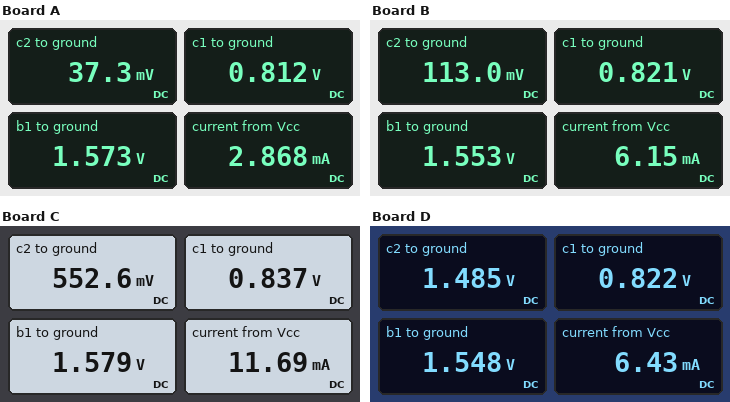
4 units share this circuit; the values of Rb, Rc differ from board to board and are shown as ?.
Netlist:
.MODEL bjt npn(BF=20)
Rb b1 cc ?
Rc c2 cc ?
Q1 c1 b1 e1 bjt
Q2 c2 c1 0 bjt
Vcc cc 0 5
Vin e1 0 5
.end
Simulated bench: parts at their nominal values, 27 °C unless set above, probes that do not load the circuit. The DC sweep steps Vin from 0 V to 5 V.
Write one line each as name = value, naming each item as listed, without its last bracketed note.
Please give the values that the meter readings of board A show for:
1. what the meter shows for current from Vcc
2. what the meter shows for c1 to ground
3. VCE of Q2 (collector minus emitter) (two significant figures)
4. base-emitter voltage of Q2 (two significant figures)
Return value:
what the meter shows for current from Vcc = 2.868 mA
what the meter shows for c1 to ground = 0.812 V
VCE of Q2 (collector minus emitter) = 37 mV
base-emitter voltage of Q2 = 810 mV
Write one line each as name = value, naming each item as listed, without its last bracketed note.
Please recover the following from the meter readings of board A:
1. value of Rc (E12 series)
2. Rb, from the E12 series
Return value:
value of Rc = 2.2 kΩ
Rb, from the E12 series = 5.6 kΩ
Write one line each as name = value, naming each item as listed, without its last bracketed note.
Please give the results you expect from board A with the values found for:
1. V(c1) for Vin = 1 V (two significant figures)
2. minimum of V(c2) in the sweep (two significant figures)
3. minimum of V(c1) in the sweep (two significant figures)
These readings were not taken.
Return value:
V(c1) for Vin = 1 V = 810 mV
minimum of V(c2) in the sweep = 37 mV
minimum of V(c1) in the sweep = 18 mV
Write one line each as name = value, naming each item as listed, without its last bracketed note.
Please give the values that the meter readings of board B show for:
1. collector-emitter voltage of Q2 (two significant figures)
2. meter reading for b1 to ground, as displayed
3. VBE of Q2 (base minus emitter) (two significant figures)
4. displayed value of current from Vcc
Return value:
collector-emitter voltage of Q2 = 110 mV
meter reading for b1 to ground, as displayed = 1.553 V
VBE of Q2 (base minus emitter) = 820 mV
displayed value of current from Vcc = 6.15 mA
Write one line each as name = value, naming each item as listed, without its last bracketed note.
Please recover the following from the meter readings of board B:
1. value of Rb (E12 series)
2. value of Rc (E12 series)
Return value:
value of Rb = 18 kΩ
value of Rc = 820 Ω
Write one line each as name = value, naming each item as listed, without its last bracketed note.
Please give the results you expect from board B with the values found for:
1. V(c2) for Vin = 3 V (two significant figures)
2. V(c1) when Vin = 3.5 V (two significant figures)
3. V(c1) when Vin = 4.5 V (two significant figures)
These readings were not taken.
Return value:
V(c2) for Vin = 3 V = 110 mV
V(c1) when Vin = 3.5 V = 820 mV
V(c1) when Vin = 4.5 V = 820 mV
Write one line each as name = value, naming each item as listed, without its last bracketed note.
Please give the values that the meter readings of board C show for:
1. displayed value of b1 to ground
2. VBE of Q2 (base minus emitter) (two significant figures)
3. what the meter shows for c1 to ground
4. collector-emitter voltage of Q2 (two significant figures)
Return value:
displayed value of b1 to ground = 1.579 V
VBE of Q2 (base minus emitter) = 840 mV
what the meter shows for c1 to ground = 0.837 V
collector-emitter voltage of Q2 = 550 mV
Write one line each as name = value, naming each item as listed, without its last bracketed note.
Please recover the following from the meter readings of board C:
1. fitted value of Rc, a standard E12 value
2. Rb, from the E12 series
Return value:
fitted value of Rc, a standard E12 value = 390 Ω
Rb, from the E12 series = 12 kΩ
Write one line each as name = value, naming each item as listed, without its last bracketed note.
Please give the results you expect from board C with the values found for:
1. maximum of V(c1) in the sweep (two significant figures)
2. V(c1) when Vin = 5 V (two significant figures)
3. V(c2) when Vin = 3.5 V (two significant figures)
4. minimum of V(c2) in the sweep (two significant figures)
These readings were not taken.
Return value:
maximum of V(c1) in the sweep = 840 mV
V(c1) when Vin = 5 V = 840 mV
V(c2) when Vin = 3.5 V = 550 mV
minimum of V(c2) in the sweep = 550 mV
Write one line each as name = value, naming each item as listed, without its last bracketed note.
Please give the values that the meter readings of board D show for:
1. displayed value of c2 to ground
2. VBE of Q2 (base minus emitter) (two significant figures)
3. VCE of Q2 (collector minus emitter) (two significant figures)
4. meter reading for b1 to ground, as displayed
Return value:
displayed value of c2 to ground = 1.485 V
VBE of Q2 (base minus emitter) = 820 mV
VCE of Q2 (collector minus emitter) = 1.5 V
meter reading for b1 to ground, as displayed = 1.548 V
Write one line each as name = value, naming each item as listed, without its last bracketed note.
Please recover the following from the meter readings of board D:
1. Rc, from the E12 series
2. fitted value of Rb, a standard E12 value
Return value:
Rc, from the E12 series = 560 Ω
fitted value of Rb, a standard E12 value = 22 kΩ
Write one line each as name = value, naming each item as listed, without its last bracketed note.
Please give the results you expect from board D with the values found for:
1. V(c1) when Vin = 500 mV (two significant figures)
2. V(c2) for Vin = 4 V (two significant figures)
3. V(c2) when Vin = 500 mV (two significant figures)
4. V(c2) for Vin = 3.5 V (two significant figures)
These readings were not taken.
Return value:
V(c1) when Vin = 500 mV = 520 mV
V(c2) for Vin = 4 V = 1.5 V
V(c2) when Vin = 500 mV = 5.0 V
V(c2) for Vin = 3.5 V = 1.5 V
